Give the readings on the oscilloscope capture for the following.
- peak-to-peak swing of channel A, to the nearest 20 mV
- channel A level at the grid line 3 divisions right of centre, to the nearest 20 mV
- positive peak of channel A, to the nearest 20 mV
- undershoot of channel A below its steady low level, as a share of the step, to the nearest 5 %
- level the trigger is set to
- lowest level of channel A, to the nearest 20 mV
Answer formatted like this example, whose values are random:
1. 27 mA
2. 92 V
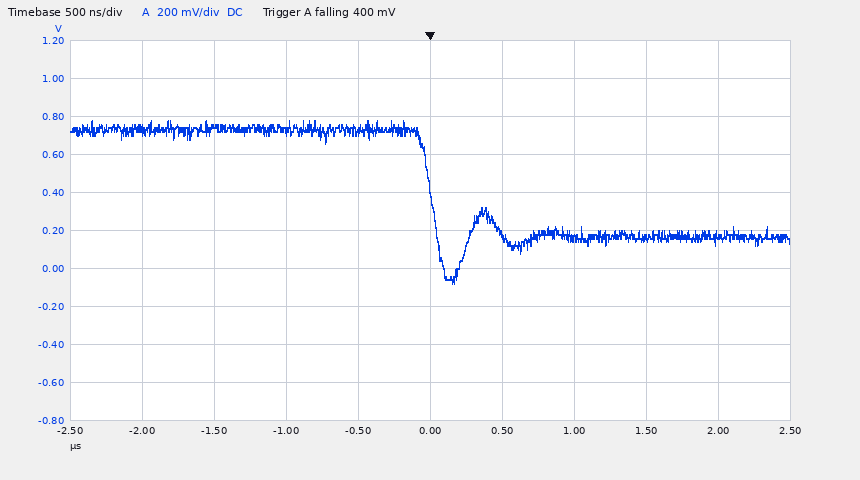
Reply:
1. 860 mV
2. 160 mV
3. 780 mV
4. 45 %
5. 400 mV
6. -80 mV
